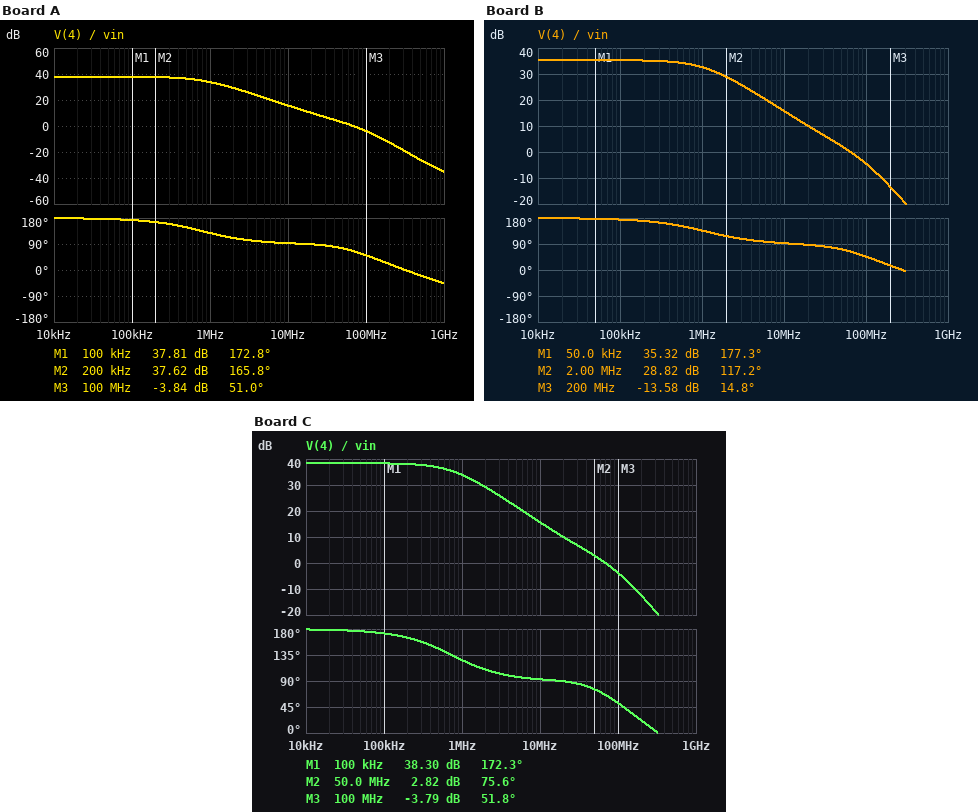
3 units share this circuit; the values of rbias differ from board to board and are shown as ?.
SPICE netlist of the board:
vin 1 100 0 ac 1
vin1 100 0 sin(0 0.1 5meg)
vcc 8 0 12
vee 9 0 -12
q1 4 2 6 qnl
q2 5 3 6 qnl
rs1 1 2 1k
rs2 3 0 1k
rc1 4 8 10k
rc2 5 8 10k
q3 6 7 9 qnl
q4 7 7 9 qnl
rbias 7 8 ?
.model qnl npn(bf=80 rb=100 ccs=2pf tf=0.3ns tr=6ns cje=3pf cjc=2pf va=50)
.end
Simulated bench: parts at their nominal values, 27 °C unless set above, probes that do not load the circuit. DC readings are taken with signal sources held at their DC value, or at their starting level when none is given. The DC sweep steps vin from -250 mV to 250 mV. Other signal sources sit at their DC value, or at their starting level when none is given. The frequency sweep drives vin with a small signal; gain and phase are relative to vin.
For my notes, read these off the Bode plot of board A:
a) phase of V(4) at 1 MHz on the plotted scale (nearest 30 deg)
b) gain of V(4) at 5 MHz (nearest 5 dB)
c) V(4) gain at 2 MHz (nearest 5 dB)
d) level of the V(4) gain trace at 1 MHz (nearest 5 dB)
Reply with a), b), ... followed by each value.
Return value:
a) 120 deg
b) 20 dB
c) 30 dB
d) 35 dB
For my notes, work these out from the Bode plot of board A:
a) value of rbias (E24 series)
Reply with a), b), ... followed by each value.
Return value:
a) 24 kΩ
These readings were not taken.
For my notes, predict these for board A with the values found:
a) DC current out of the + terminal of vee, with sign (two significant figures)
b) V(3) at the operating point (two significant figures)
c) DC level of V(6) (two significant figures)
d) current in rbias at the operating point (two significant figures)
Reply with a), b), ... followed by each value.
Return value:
a) -2.1 mA
b) -6.3 mV
c) -760 mV
d) 970 µA
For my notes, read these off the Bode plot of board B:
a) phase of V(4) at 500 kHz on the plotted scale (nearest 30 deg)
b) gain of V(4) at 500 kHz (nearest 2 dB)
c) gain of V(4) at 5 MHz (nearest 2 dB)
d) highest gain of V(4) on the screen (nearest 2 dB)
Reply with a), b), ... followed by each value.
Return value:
a) 150 deg
b) 34 dB
c) 22 dB
d) 36 dB
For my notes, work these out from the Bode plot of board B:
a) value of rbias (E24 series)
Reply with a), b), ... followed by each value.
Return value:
a) 36 kΩ
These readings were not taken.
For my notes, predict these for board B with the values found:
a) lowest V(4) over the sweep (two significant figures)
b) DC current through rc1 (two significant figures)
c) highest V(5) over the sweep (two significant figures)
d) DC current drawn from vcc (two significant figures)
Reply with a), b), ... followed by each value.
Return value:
a) 4.4 V
b) 380 µA
c) 12 V
d) 1.4 mA
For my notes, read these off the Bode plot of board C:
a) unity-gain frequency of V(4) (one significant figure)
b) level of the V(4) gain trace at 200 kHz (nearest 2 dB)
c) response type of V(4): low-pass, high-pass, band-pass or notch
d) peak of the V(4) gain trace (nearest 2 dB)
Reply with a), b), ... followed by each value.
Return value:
a) 70 MHz
b) 38 dB
c) low-pass
d) 38 dB
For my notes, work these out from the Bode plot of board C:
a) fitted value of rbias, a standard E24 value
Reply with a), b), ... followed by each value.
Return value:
a) 22 kΩ
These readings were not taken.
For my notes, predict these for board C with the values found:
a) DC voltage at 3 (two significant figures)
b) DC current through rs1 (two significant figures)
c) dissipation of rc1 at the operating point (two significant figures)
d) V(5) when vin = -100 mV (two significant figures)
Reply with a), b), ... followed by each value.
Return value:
a) -6.9 mV
b) 6.9 µA
c) 3.8 mW
d) 250 mV
